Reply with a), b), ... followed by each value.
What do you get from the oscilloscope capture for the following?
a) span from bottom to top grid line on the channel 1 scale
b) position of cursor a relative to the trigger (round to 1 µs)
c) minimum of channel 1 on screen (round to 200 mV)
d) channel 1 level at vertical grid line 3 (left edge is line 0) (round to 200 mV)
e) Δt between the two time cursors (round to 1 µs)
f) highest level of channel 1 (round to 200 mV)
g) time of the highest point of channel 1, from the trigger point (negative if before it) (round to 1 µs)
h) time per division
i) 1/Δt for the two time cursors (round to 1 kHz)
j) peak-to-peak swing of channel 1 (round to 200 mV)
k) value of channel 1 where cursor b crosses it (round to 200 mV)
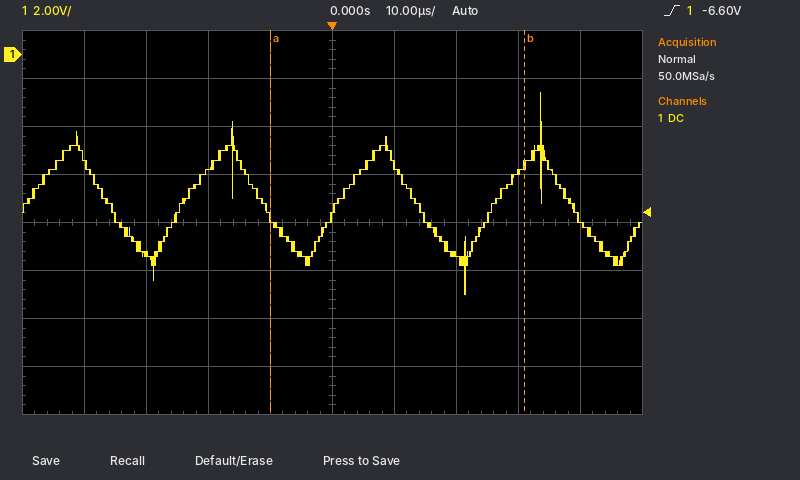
a) 16 V
b) -10 µs
c) -10.0 V
d) -4.8 V
e) 41 µs
f) -1.6 V
g) +34 µs
h) 10 µs
i) 24 kHz
j) 8.4 V
k) -4.6 V
